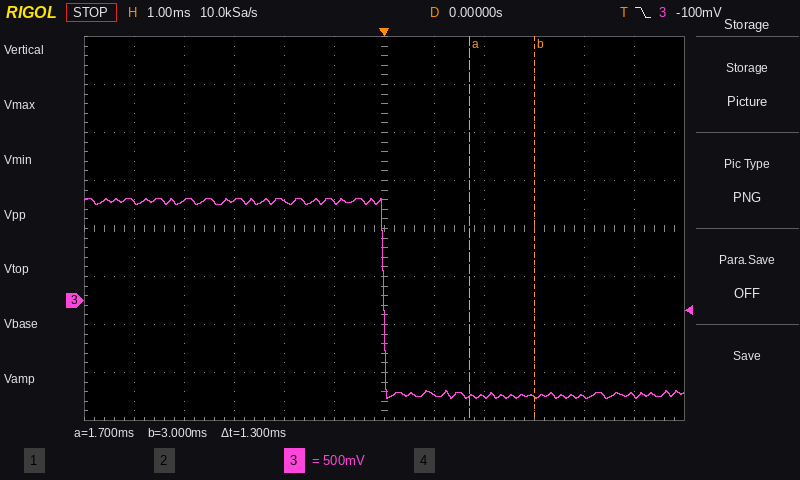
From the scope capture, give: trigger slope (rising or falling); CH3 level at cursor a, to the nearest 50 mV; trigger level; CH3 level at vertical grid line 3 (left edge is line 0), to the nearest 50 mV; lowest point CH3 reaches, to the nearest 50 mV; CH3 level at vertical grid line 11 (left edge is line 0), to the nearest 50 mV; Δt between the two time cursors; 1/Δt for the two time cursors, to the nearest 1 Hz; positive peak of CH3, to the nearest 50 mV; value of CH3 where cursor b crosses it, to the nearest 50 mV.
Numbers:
falling
-1.00 V
-100 mV
1.05 V
-1.00 V
-1.00 V
1.3 ms
769 Hz
1.05 V
-1.00 V
